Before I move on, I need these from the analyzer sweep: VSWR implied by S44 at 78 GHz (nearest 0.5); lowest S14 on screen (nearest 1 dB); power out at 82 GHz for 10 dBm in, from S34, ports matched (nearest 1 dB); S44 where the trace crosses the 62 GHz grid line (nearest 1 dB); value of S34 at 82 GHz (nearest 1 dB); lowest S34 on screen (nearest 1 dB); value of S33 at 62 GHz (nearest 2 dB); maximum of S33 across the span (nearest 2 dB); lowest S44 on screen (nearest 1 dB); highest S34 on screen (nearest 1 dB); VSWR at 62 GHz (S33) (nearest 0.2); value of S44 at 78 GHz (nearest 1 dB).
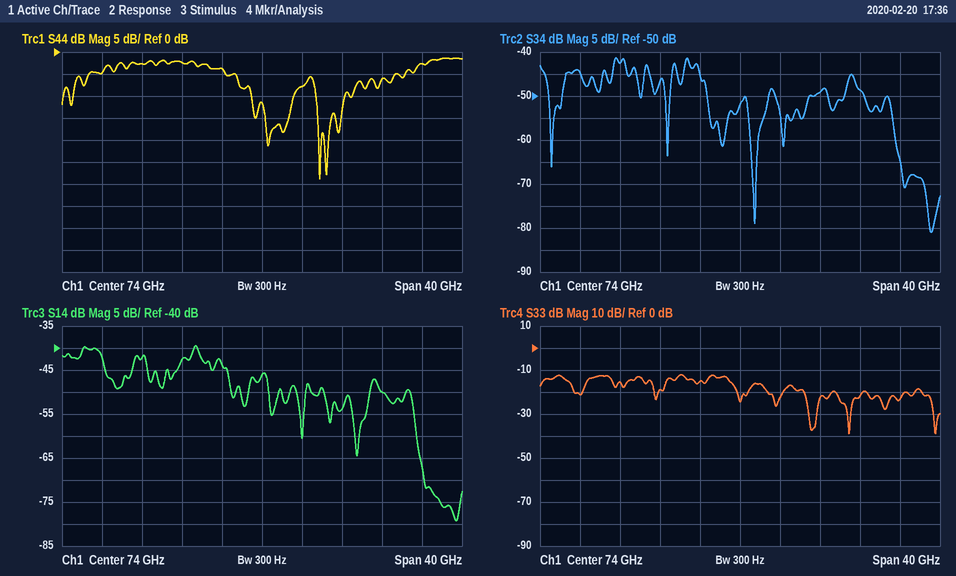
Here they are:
2.5
-79 dB
-39 dBm
-3 dB
-49 dB
-81 dB
-16 dB
-12 dB
-29 dB
-41 dB
1.4
-8 dB
